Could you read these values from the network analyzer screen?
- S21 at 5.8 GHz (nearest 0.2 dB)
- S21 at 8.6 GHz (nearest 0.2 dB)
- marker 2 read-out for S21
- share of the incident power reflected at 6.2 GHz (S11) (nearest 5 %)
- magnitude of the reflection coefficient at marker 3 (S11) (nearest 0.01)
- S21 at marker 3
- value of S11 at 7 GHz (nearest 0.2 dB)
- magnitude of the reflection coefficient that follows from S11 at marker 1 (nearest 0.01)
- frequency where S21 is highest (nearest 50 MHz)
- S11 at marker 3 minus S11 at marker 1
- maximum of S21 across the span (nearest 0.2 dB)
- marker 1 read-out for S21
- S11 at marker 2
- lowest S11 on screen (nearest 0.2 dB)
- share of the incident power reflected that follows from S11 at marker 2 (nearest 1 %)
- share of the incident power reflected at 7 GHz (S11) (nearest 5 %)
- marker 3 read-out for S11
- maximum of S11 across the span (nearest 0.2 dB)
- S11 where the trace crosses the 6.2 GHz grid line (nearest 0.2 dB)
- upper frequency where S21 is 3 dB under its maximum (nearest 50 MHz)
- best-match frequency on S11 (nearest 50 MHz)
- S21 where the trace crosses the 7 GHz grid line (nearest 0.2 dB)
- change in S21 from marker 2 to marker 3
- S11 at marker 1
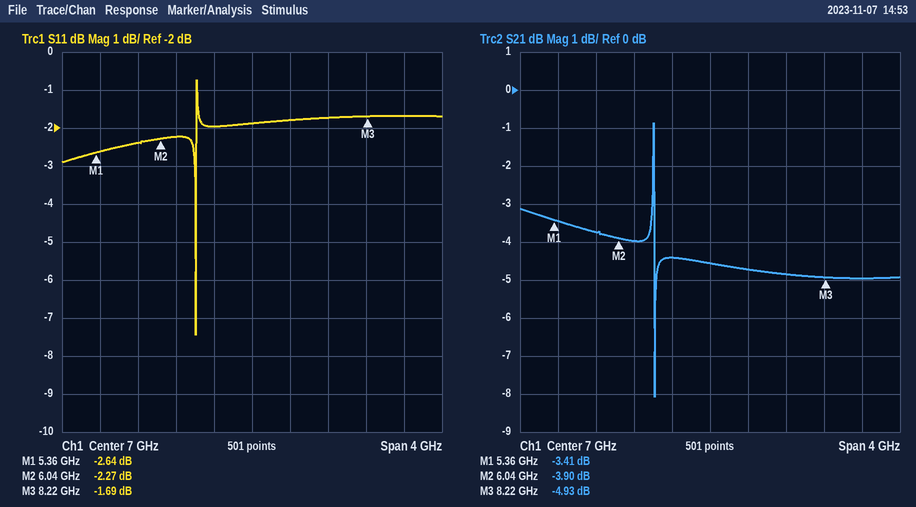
-3.8 dB
-5.0 dB
-3.90 dB
60 %
0.82
-4.93 dB
-1.8 dB
0.74
6.40 GHz
0.95 dB
-0.8 dB
-3.41 dB
-2.27 dB
-7.4 dB
59 %
65 %
-1.69 dB
-0.8 dB
-2.2 dB
6.40 GHz
6.40 GHz
-4.6 dB
-1.03 dB
-2.64 dB
